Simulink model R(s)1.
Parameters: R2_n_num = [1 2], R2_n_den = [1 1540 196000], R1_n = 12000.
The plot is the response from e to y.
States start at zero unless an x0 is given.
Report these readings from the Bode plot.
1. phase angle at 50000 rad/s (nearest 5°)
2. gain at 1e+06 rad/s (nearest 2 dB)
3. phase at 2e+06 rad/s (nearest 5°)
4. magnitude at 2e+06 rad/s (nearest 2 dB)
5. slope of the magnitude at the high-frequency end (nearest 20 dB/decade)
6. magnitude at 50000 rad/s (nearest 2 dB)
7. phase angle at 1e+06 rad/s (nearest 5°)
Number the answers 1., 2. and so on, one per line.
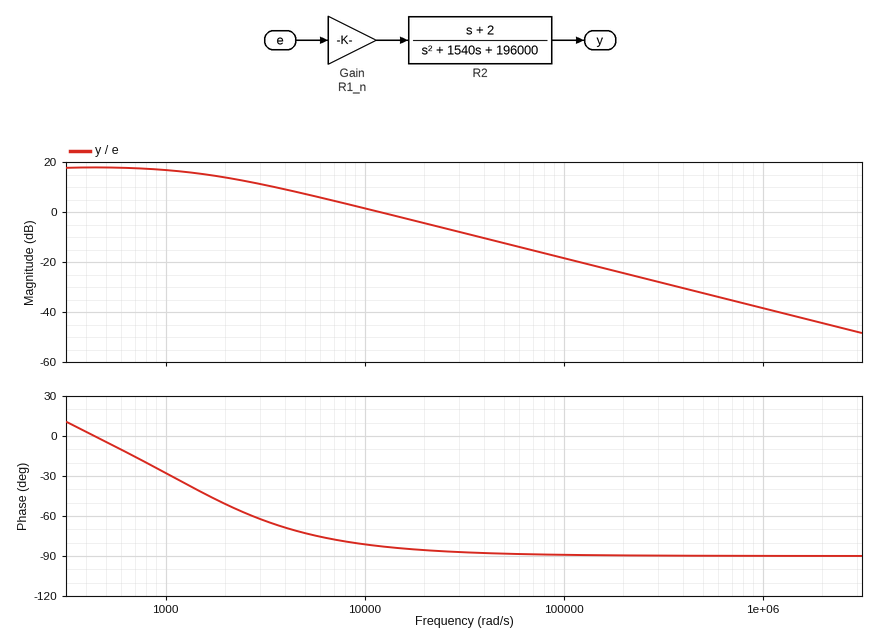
1. -90°
2. -38 dB
3. -90°
4. -44 dB
5. -20 dB/decade
6. -12 dB
7. -90°
